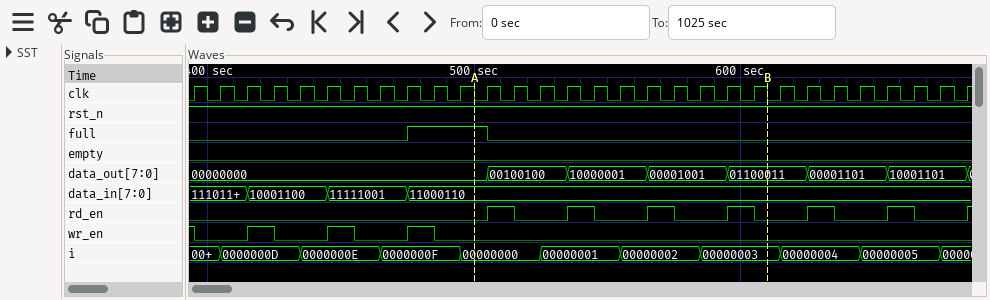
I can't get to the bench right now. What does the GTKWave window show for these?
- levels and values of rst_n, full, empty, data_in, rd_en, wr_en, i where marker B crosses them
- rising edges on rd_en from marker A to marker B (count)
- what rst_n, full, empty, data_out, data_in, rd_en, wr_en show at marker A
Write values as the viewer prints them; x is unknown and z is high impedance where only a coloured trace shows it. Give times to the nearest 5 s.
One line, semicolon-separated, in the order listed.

rst_n=1, full=0, empty=0, data_in=11000110, rd_en=0, wr_en=0, i=00000003; 4; rst_n=1, full=1, empty=0, data_out=00000000, data_in=11000110, rd_en=0, wr_en=0
